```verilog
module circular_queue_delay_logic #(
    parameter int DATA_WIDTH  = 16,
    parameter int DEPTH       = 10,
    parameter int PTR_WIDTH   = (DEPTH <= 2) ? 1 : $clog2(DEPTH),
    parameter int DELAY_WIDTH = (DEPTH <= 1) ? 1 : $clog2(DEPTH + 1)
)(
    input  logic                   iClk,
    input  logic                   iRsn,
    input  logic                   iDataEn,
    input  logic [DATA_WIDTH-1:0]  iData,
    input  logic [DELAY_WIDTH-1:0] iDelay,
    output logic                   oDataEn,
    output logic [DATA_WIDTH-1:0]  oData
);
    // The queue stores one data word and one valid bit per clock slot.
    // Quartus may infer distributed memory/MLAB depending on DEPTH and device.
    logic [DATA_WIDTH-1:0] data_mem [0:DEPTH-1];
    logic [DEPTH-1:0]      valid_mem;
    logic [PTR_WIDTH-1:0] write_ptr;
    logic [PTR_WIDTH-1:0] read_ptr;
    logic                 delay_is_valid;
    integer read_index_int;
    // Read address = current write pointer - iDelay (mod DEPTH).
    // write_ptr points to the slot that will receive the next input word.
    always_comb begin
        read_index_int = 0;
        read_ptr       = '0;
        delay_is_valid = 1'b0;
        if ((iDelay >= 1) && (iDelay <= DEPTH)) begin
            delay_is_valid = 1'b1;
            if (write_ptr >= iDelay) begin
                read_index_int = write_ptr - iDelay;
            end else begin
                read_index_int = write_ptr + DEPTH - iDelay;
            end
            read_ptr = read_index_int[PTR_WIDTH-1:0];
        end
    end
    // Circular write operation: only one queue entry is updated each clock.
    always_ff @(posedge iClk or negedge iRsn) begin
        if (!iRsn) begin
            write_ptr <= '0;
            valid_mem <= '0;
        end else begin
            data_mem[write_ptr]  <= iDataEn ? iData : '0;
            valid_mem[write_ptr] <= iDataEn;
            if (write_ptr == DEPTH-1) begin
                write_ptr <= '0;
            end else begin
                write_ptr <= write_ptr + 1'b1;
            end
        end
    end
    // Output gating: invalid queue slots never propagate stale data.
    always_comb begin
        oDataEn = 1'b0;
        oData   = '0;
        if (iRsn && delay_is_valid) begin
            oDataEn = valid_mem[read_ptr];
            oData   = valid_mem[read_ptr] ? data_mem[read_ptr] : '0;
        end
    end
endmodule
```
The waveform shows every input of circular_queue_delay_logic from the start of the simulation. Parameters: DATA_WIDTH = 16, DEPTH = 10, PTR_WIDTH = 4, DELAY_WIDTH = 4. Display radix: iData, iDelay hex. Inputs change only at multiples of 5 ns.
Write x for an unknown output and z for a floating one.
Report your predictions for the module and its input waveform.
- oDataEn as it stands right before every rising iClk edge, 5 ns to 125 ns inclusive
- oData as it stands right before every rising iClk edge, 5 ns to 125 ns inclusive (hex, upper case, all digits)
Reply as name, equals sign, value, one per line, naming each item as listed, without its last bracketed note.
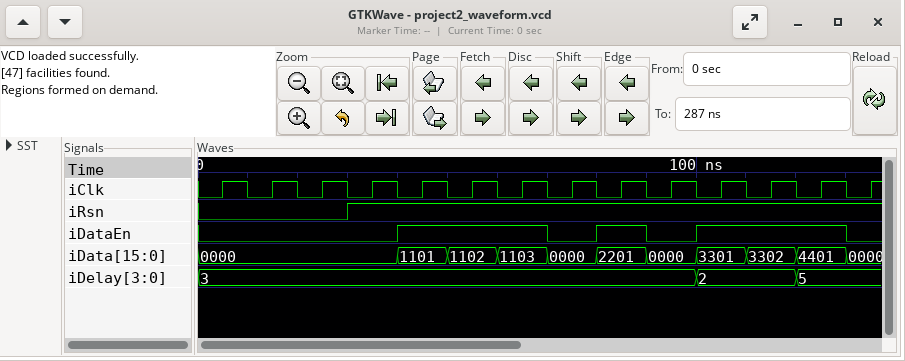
oDataEn as it stands right before every rising iClk edge, 5 ns to 125 ns inclusive = 0 0 0 0 0 0 0 1 1 1 1 0 0
oData as it stands right before every rising iClk edge, 5 ns to 125 ns inclusive = 0000, 0000, 0000, 0000, 0000, 0000, 0000, 1101, 1102, 1103, 2201, 0000, 0000
